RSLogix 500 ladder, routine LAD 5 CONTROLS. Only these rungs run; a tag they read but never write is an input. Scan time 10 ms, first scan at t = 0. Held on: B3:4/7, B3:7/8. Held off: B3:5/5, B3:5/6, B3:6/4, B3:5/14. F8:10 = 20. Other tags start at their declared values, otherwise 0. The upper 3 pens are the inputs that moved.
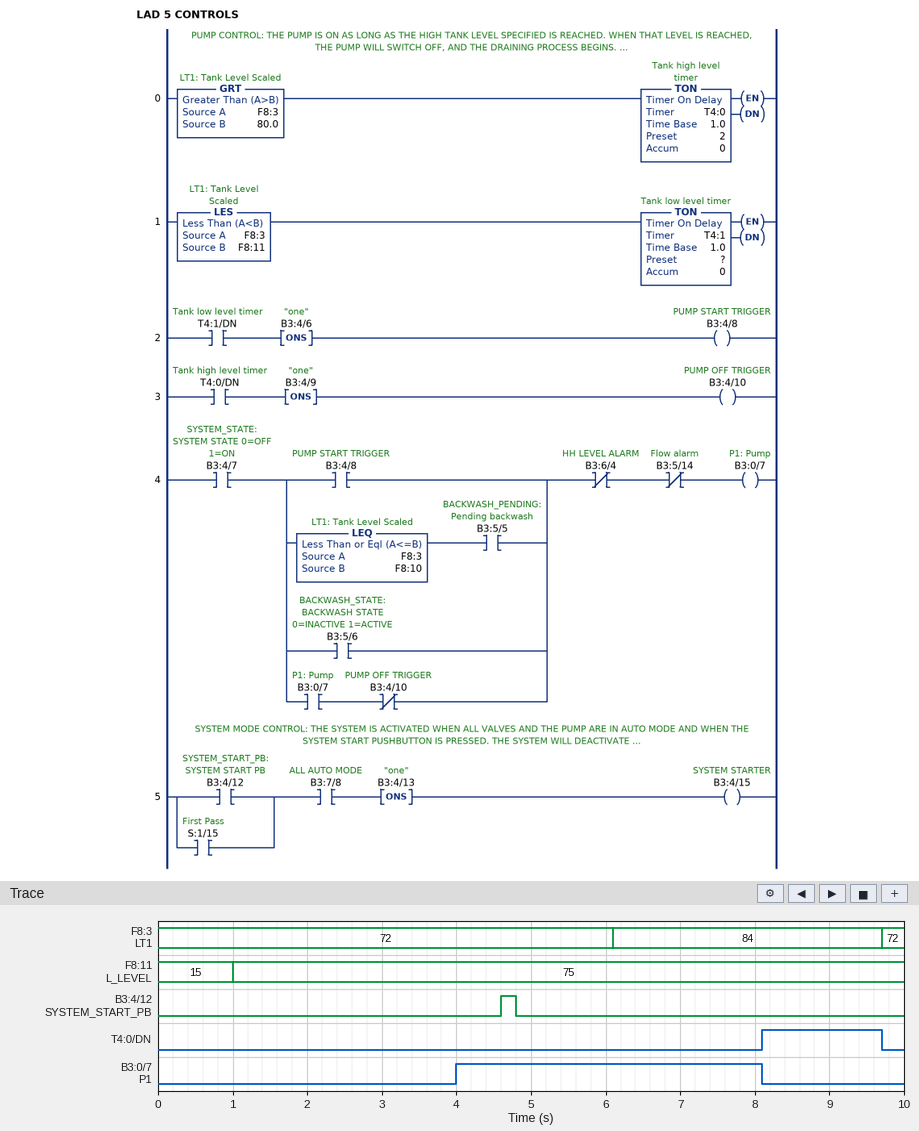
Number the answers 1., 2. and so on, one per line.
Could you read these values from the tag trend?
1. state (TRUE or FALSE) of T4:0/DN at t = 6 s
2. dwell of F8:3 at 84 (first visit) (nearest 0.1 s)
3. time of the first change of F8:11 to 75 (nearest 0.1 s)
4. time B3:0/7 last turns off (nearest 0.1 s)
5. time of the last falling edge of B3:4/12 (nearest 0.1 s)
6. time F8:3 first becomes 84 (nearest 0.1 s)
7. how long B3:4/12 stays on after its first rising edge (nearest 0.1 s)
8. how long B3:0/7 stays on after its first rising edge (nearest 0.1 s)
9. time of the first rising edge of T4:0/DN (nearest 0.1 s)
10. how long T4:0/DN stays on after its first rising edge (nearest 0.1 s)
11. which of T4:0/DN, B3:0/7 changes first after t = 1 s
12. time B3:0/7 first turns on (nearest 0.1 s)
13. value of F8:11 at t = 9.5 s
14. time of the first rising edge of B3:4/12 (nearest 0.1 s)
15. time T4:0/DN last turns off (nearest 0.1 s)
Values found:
1. FALSE
2. 3.6 s
3. 1.0 s
4. 8.1 s
5. 4.8 s
6. 6.1 s
7. 0.2 s
8. 4.1 s
9. 8.1 s
10. 1.6 s
11. B3:0/7
12. 4.0 s
13. 75
14. 4.6 s
15. 9.7 s
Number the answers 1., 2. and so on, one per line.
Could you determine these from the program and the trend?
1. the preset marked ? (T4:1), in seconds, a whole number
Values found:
1. 3 s
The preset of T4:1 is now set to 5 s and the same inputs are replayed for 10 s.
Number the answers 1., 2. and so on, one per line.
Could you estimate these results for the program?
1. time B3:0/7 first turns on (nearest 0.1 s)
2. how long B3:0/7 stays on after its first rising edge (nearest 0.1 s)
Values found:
1. 6.0 s
2. 2.1 s
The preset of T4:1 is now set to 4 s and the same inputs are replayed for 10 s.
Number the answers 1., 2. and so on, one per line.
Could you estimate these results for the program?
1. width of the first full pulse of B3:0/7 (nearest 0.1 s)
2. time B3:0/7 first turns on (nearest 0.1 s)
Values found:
1. 3.1 s
2. 5.0 s
